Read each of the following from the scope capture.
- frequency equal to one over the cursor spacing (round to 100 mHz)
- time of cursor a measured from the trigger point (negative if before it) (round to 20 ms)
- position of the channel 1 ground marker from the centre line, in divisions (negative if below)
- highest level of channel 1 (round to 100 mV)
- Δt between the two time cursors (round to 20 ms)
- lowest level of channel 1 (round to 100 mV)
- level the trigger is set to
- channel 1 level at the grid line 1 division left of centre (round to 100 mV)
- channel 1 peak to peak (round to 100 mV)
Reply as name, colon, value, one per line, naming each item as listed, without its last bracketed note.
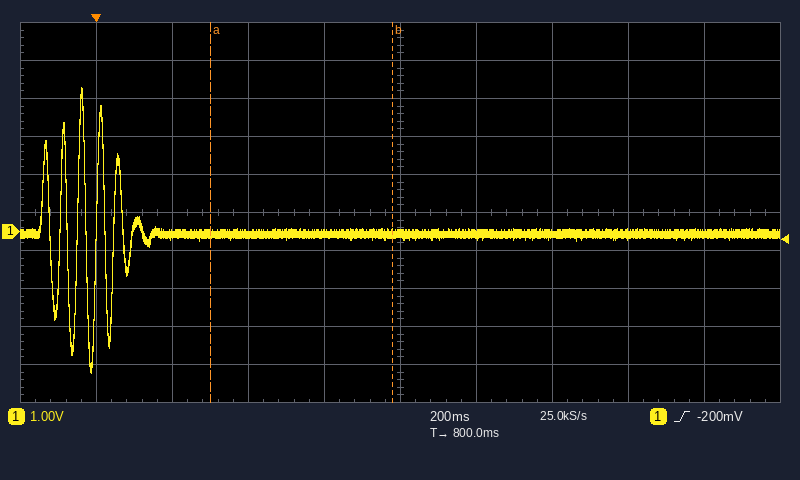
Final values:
frequency equal to one over the cursor spacing: 2.1 Hz
time of cursor a measured from the trigger point (negative if before it): +300 ms
position of the channel 1 ground marker from the centre line, in divisions: -0.5 div
highest level of channel 1: 3.8 V
Δt between the two time cursors: 480 ms
lowest level of channel 1: -3.7 V
level the trigger is set to: -200 mV
channel 1 level at the grid line 1 division left of centre: -100 mV
channel 1 peak to peak: 7.5 V
